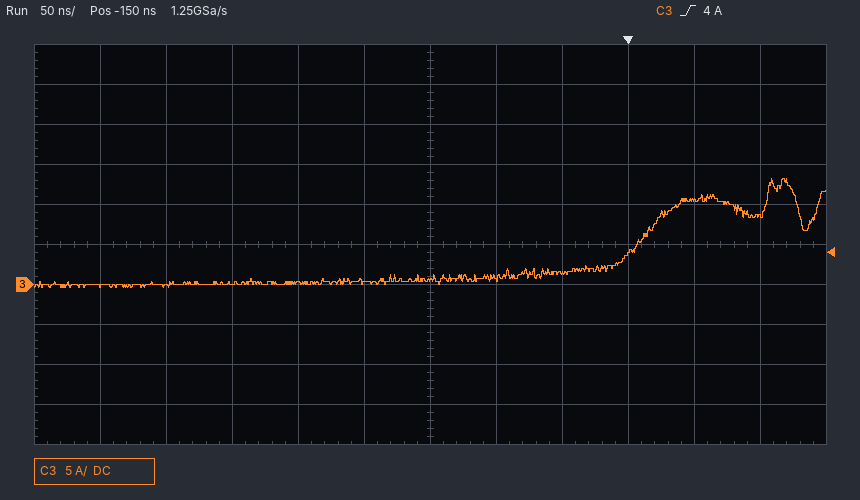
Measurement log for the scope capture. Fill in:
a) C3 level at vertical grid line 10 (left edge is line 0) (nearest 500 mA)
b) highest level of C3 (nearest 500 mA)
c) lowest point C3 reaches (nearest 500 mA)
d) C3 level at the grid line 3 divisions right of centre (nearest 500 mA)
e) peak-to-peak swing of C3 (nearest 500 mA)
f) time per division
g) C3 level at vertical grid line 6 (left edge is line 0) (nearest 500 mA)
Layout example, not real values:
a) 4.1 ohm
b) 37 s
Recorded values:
a) 10.5 A
b) 13.0 A
c) -500 mA
d) 4.0 A
e) 13.5 A
f) 50 ns
g) 500 mA
